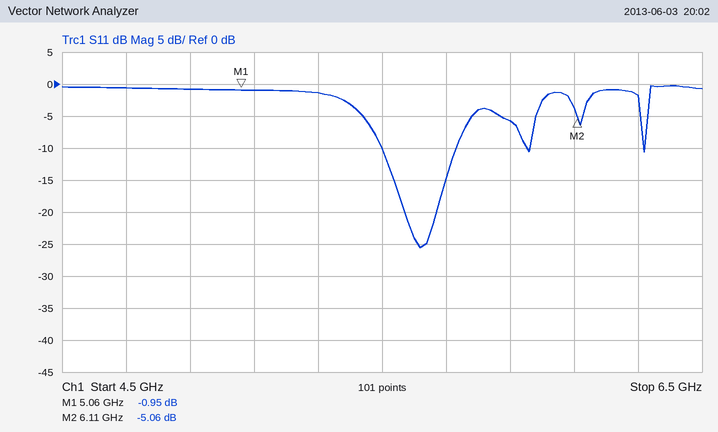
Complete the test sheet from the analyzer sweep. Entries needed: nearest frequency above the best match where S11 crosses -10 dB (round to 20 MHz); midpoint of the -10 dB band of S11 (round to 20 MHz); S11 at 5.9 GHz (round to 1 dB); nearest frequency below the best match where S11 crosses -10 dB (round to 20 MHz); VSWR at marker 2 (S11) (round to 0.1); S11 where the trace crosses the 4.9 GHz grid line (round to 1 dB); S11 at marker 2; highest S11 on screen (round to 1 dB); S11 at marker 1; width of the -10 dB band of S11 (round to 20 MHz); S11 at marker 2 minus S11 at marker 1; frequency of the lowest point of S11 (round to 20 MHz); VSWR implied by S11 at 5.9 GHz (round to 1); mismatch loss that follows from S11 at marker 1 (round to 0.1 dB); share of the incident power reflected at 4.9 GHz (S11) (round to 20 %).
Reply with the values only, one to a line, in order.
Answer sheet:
5.74 GHz
5.62 GHz
-6 dB
5.50 GHz
3.5
-1 dB
-5.06 dB
0 dB
-0.95 dB
240 MHz
-4.11 dB
5.62 GHz
3
7.1 dB
80 %
